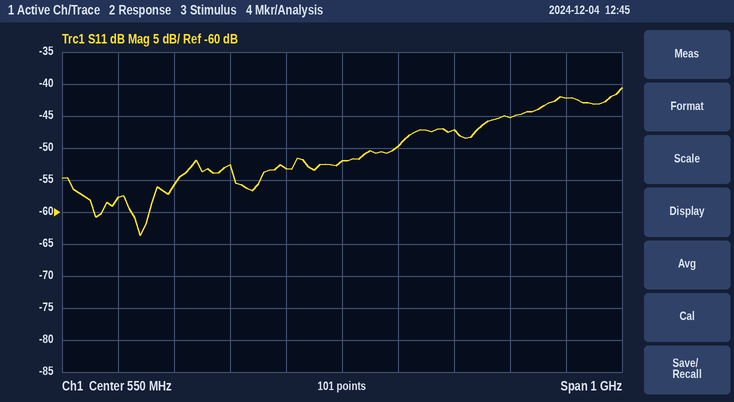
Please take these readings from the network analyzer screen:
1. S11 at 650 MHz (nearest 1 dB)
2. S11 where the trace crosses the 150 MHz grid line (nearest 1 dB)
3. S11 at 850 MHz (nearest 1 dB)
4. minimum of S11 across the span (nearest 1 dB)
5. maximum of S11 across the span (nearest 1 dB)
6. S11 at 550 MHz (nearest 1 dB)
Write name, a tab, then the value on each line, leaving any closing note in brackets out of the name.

S11 at 650 MHz	-50 dB
S11 where the trace crosses the 150 MHz grid line	-58 dB
S11 at 850 MHz	-45 dB
minimum of S11 across the span	-64 dB
maximum of S11 across the span	-41 dB
S11 at 550 MHz	-52 dB
